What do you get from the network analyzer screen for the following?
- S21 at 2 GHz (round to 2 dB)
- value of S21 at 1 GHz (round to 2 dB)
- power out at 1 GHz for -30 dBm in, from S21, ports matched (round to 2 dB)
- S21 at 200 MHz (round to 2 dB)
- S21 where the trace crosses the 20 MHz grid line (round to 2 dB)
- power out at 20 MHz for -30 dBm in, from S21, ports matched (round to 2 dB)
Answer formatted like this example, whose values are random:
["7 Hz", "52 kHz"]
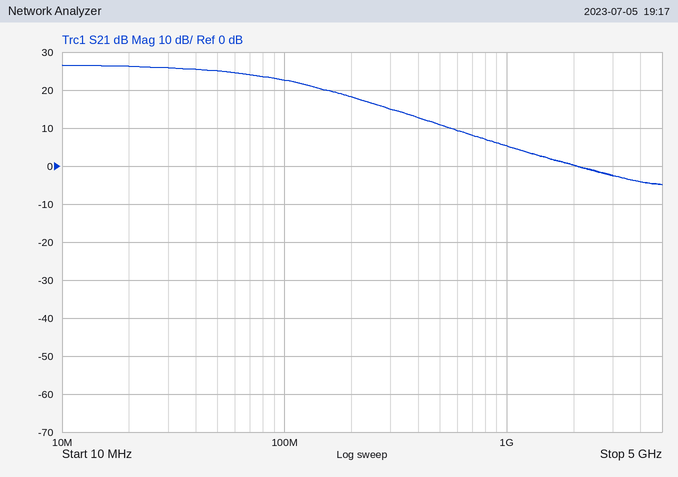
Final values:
["0 dB", "6 dB", "-24 dBm", "18 dB", "26 dB", "-4 dBm"]
